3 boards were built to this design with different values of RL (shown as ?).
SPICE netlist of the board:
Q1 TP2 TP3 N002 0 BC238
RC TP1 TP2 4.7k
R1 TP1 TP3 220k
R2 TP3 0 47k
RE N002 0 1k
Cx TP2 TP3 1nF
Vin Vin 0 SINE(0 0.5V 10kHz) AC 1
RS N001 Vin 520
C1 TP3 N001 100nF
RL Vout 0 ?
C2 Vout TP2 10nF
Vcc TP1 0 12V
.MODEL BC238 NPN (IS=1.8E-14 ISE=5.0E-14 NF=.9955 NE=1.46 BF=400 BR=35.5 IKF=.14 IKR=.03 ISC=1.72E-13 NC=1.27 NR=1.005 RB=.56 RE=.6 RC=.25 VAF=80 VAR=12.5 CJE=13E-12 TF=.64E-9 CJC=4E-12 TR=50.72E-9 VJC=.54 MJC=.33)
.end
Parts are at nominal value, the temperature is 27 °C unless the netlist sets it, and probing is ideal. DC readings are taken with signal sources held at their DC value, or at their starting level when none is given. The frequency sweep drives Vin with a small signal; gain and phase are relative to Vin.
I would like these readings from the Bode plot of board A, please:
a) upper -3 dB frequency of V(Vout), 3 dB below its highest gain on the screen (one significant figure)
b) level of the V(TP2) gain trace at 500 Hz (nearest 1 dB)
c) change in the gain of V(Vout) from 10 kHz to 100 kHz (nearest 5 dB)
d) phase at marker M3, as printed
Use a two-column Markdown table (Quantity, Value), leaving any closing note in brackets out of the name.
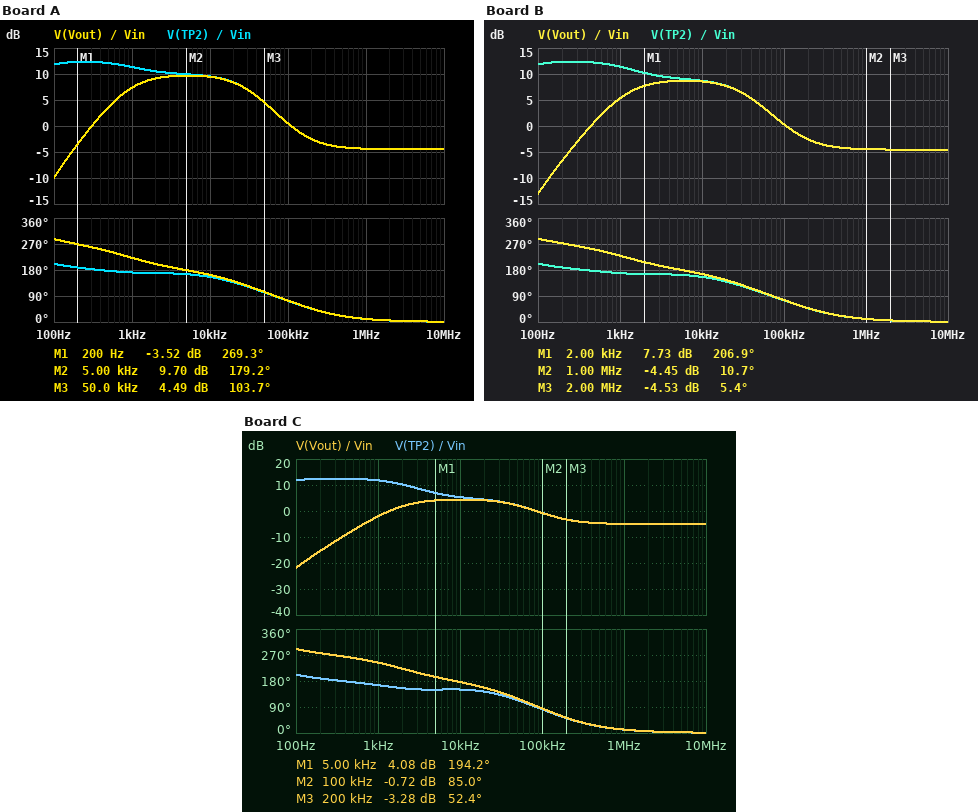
| Quantity | Value |
|---|---|
| upper -3 dB frequency of V(Vout), 3 dB below its highest gain on the screen | 30 kHz |
| level of the V(TP2) gain trace at 500 Hz | 12 dB |
| change in the gain of V(Vout) from 10 kHz to 100 kHz | -10 dB |
| phase at marker M3, as printed | 103.7 deg |
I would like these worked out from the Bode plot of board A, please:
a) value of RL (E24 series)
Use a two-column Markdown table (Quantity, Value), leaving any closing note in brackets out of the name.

| Quantity | Value |
|---|---|
| value of RL | 13 kΩ |
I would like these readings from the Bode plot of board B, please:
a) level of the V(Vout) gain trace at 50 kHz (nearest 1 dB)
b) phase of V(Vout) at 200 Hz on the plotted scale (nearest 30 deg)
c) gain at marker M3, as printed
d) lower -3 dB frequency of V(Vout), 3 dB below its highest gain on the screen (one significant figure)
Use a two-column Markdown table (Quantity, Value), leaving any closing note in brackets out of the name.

| Quantity | Value |
|---|---|
| level of the V(Vout) gain trace at 50 kHz | 4 dB |
| phase of V(Vout) at 200 Hz on the plotted scale | 270 deg |
| gain at marker M3, as printed | -4.53 dB |
| lower -3 dB frequency of V(Vout), 3 dB below its highest gain on the screen | 1 kHz |
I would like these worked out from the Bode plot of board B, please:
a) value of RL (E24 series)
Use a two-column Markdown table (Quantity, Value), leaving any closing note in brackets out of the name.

| Quantity | Value |
|---|---|
| value of RL | 9.1 kΩ |
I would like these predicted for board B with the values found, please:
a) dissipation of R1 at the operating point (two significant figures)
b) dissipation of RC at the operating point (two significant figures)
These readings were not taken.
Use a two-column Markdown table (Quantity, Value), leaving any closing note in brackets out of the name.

| Quantity | Value |
|---|---|
| dissipation of R1 at the operating point | 460 µW |
| dissipation of RC at the operating point | 7.8 mW |
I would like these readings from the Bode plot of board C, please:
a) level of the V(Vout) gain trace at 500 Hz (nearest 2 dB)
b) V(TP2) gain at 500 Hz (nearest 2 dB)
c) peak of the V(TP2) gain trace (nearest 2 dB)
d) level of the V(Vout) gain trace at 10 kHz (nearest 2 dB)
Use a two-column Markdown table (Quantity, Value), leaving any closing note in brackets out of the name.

| Quantity | Value |
|---|---|
| level of the V(Vout) gain trace at 500 Hz | -8 dB |
| V(TP2) gain at 500 Hz | 12 dB |
| peak of the V(TP2) gain trace | 12 dB |
| level of the V(Vout) gain trace at 10 kHz | 4 dB |
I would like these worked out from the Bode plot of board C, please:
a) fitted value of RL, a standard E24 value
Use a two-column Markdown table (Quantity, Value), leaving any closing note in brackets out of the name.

| Quantity | Value |
|---|---|
| fitted value of RL, a standard E24 value | 3.3 kΩ |
